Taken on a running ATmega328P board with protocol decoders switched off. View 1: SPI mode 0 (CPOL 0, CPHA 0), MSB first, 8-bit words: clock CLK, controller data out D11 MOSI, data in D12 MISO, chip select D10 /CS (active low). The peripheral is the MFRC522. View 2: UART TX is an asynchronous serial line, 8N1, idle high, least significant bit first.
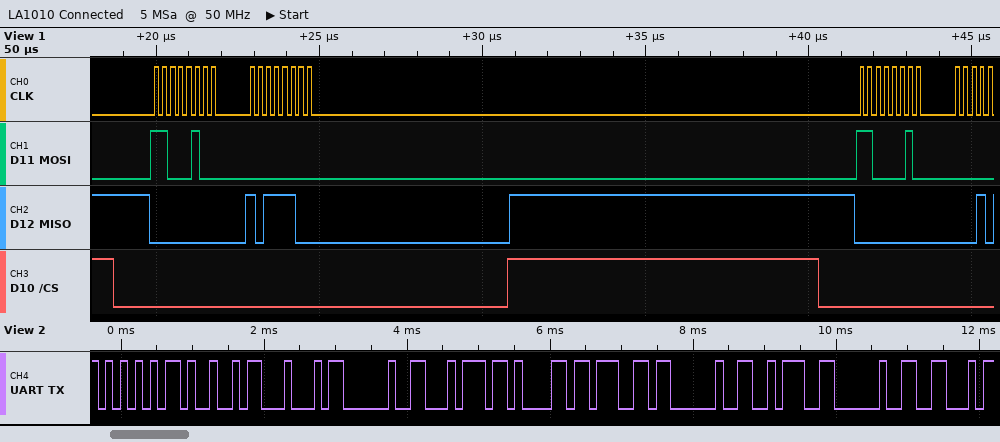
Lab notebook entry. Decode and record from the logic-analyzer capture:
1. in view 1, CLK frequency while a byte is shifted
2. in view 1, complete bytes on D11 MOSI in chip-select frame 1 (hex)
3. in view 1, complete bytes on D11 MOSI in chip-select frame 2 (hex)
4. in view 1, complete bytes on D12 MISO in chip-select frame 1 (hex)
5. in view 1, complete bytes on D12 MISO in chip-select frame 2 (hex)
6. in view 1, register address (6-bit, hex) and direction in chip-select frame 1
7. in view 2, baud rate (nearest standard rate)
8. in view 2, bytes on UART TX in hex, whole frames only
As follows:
4 MHz
C4 00
C2
00 BC
00
0x22 read
9600 baud
55 49 44 20 74 61 67 20 3A 20 46
